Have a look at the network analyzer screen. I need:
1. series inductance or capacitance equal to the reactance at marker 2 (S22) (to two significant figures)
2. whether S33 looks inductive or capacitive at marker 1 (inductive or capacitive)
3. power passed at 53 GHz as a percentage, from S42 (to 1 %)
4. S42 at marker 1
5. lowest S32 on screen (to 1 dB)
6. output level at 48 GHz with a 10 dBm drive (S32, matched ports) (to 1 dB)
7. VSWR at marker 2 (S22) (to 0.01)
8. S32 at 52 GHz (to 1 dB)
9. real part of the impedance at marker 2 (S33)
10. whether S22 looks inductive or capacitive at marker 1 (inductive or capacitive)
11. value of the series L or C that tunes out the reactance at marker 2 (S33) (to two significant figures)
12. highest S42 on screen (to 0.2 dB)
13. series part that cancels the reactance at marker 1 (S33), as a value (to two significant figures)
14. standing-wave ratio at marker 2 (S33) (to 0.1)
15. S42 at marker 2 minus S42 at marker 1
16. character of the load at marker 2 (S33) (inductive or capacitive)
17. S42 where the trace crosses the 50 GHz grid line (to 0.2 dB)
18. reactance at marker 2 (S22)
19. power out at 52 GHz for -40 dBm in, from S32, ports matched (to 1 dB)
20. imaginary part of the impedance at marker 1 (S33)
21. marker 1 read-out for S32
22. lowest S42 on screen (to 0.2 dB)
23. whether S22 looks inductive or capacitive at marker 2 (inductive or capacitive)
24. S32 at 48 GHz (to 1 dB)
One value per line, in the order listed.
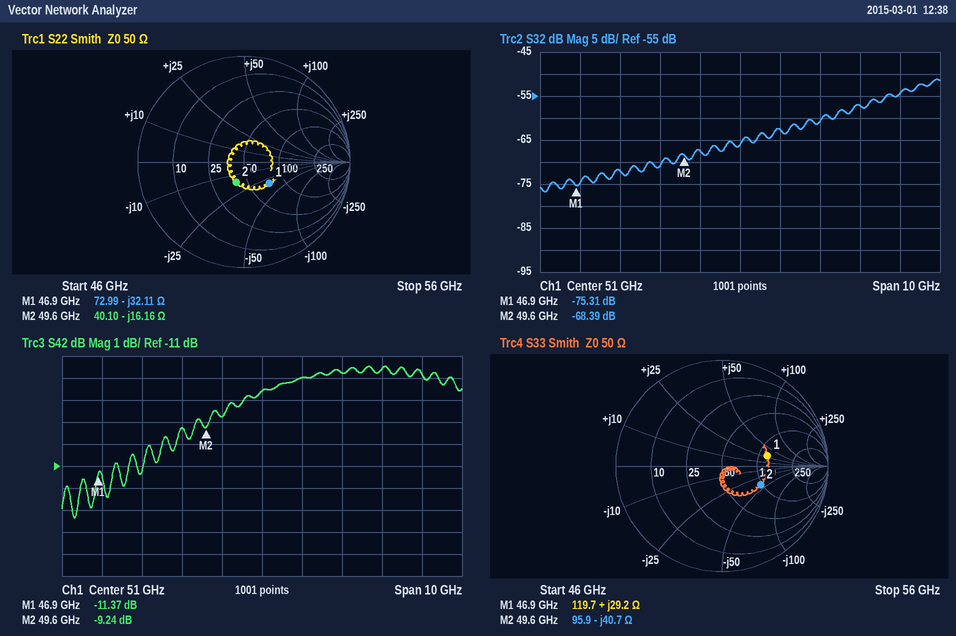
200 fF
inductive
21 %
-11.37 dB
-77 dB
-62 dBm
1.52
-63 dB
95.9 Ω
capacitive
130 pH
-6.4 dB
120 fF
2.4
2.13 dB
capacitive
-8.8 dB
-16.16 Ω
-103 dBm
+29.2 Ω
-75.31 dB
-13.4 dB
capacitive
-72 dB
